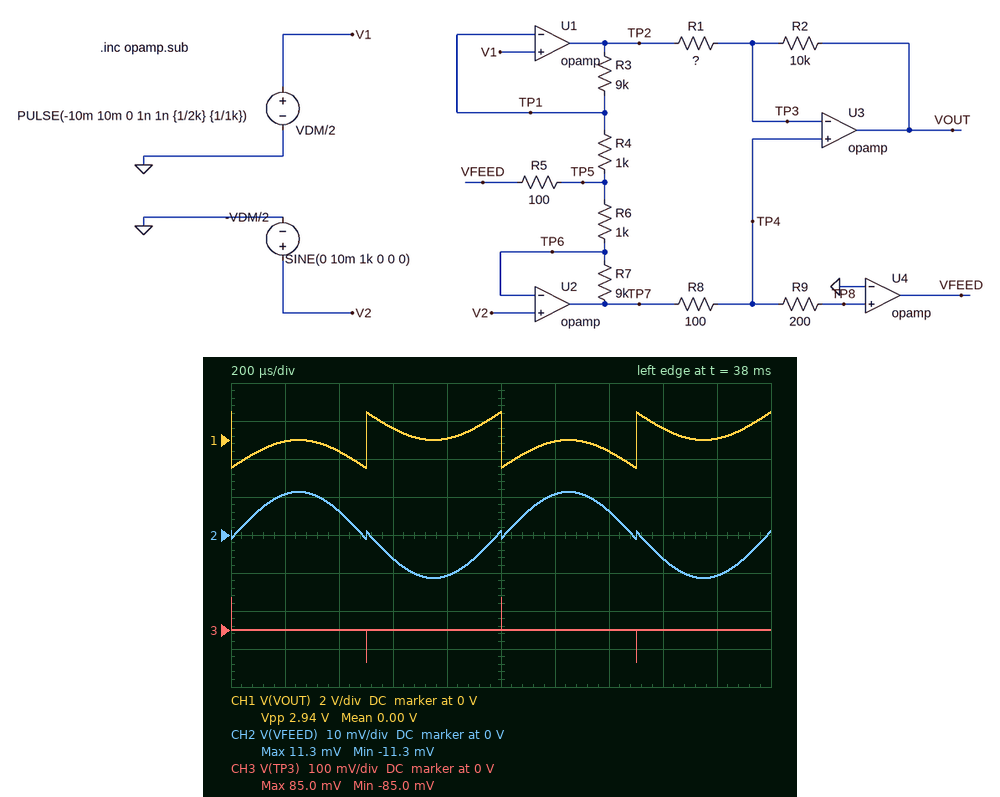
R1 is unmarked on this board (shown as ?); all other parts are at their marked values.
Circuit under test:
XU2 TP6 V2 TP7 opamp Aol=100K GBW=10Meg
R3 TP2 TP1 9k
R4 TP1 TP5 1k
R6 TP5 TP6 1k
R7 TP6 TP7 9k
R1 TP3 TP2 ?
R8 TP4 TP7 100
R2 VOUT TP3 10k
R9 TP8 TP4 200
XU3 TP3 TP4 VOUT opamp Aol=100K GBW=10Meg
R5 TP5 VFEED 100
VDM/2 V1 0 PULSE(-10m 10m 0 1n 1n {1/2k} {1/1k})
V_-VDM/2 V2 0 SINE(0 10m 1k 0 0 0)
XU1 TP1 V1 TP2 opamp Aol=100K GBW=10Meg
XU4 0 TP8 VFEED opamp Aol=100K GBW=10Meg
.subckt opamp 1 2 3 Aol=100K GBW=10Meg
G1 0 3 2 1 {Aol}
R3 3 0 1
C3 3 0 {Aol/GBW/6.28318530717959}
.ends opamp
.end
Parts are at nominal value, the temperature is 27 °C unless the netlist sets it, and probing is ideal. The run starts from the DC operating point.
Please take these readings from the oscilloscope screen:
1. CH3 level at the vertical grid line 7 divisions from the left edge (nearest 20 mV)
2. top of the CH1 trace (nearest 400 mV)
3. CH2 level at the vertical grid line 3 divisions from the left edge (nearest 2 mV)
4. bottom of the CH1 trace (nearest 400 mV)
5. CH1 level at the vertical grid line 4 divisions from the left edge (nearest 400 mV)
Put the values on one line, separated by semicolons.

0 V; 1.6 V; -6 mV; -1.6 V; 0 V
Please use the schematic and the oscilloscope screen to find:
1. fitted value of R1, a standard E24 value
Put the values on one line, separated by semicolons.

680 Ω
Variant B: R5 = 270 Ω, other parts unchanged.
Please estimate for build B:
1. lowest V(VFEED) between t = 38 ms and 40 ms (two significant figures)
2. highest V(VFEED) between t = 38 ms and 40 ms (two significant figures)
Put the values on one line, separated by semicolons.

-12 mV; 12 mV
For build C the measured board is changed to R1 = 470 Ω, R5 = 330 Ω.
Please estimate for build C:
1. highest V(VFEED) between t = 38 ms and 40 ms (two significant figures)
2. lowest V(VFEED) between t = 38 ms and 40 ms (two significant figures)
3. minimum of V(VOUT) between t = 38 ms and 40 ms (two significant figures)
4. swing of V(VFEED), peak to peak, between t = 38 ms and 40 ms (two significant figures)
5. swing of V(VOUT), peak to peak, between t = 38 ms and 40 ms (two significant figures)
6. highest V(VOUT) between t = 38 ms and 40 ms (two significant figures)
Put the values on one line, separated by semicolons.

12 mV; -12 mV; -2.1 V; 24 mV; 4.2 V; 2.1 V
